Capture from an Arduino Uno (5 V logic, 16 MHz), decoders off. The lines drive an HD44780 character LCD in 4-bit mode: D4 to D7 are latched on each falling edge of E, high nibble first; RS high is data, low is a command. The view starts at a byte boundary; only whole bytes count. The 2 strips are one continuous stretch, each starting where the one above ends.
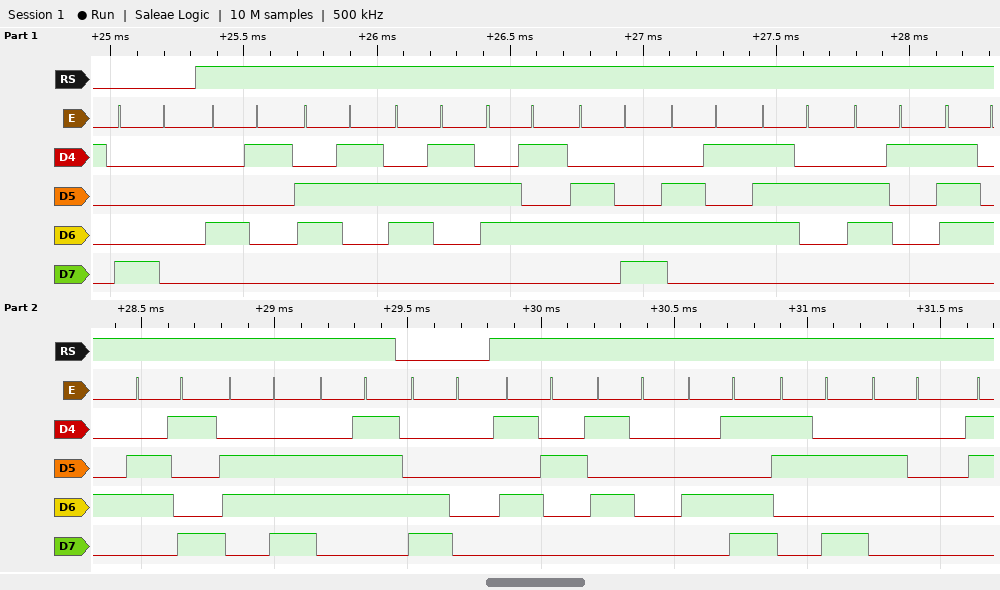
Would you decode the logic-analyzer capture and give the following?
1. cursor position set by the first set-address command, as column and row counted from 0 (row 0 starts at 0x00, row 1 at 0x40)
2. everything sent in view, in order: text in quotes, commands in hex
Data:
column 0, row 0
0x80 "Accelerating" 0xC0 "RPM: "
